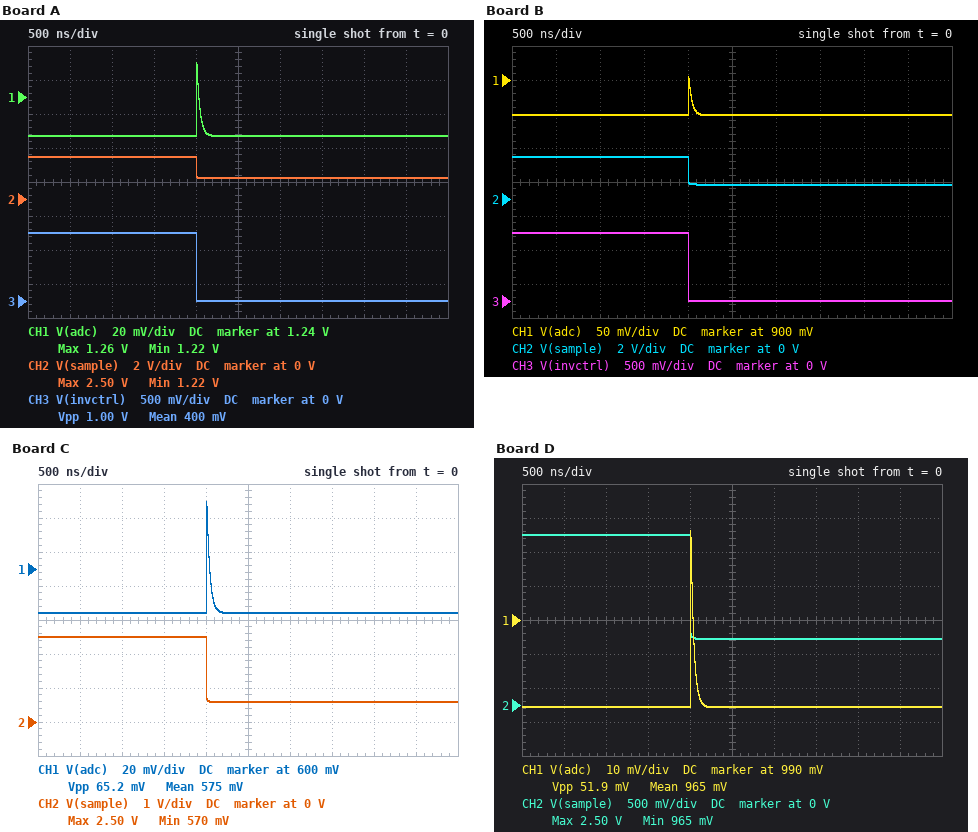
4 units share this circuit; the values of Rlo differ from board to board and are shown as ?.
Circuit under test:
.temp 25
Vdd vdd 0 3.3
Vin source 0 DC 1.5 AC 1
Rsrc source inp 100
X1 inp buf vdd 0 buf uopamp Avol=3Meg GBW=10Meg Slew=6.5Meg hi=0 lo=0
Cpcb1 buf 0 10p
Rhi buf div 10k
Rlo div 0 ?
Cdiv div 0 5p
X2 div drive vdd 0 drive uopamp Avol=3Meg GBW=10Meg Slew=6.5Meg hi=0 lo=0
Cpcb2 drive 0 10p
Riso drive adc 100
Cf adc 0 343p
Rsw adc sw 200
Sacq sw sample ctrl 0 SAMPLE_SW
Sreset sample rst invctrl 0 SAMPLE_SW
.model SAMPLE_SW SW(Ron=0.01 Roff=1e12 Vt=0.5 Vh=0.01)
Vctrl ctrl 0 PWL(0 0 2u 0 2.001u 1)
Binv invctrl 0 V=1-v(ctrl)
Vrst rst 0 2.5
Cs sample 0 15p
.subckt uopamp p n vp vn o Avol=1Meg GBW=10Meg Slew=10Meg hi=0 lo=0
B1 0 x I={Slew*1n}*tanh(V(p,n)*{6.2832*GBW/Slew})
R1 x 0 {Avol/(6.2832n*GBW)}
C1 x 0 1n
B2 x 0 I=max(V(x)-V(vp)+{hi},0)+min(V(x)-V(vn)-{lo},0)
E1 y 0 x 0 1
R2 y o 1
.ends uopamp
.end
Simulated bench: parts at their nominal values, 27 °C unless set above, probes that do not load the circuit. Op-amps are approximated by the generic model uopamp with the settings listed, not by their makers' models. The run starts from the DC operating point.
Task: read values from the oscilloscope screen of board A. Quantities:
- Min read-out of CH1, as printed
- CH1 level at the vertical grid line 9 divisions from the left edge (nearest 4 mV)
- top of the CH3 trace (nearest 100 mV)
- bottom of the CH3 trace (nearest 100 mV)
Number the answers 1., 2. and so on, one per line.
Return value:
1. 1.22 V
2. 1.216 V
3. 1.0 V
4. 0 V
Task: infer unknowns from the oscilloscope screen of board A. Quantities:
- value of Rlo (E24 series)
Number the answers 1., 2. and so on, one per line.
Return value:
1. 43 kΩ
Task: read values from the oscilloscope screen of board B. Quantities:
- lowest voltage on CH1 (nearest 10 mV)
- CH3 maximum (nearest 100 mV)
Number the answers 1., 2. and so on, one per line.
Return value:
1. 850 mV
2. 1.0 V
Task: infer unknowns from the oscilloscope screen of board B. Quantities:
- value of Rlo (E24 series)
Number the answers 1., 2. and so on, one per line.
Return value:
1. 13 kΩ
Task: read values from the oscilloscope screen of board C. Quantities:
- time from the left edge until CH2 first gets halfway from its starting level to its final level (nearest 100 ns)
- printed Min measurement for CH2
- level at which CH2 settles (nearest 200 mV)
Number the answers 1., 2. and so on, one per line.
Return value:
1. 2.0 µs
2. 570 mV
3. 600 mV
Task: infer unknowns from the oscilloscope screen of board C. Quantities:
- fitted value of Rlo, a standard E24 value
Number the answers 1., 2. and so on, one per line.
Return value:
1. 6.2 kΩ
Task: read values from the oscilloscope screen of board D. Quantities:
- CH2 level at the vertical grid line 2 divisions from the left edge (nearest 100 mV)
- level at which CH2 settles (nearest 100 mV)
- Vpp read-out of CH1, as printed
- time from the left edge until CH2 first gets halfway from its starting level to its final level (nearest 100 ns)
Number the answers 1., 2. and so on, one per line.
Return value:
1. 2.5 V
2. 1.0 V
3. 51.9 mV
4. 2.0 µs
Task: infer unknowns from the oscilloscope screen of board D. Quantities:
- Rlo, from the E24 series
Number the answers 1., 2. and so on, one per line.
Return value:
1. 18 kΩ
